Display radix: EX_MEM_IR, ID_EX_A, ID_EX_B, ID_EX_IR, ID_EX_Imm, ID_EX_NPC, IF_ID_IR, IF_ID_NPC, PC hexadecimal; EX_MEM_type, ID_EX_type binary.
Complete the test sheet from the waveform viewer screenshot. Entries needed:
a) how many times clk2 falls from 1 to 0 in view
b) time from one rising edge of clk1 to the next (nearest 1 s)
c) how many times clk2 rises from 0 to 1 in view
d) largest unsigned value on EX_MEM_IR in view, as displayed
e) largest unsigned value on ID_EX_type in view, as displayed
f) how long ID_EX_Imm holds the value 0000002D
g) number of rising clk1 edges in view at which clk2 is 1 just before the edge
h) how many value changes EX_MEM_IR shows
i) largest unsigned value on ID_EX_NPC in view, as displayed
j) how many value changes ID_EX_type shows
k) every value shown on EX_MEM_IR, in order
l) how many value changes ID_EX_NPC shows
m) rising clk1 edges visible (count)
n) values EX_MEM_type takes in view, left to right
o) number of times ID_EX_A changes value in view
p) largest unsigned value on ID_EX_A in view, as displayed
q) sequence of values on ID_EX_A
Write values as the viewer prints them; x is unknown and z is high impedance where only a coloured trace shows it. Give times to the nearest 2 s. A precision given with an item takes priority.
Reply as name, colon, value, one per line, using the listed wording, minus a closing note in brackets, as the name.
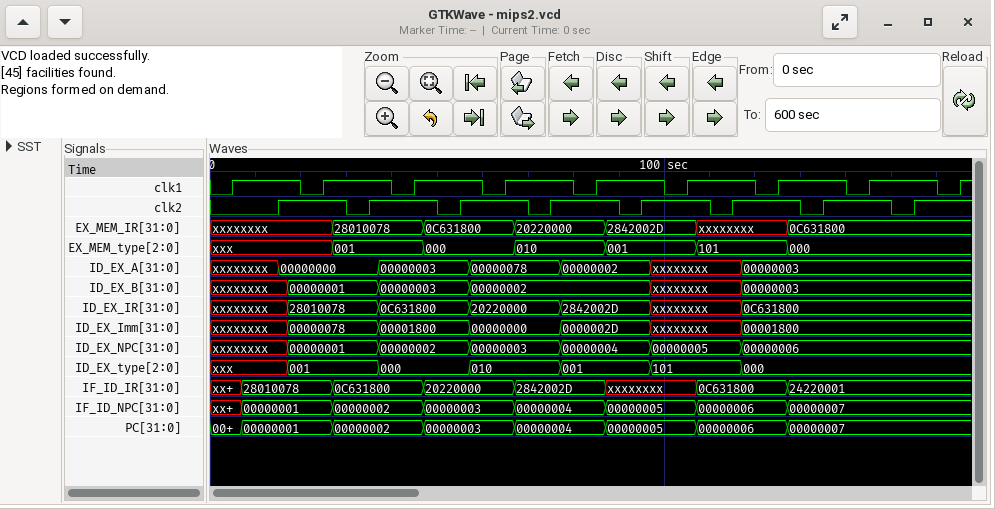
how many times clk2 falls from 1 to 0 in view: 7
time from one rising edge of clk1 to the next: 20 s
how many times clk2 rises from 0 to 1 in view: 8
largest unsigned value on EX_MEM_IR in view, as displayed: 2842002D
largest unsigned value on ID_EX_type in view, as displayed: 101
how long ID_EX_Imm holds the value 0000002D: 20 s
number of rising clk1 edges in view at which clk2 is 1 just before the edge: 8
how many value changes EX_MEM_IR shows: 6
largest unsigned value on ID_EX_NPC in view, as displayed: 00000006
how many value changes ID_EX_type shows: 6
every value shown on EX_MEM_IR, in order: xxxxxxxx, 28010078, 0C631800, 20220000, 2842002D, xxxxxxxx, 0C631800
how many value changes ID_EX_NPC shows: 6
rising clk1 edges visible: 9
values EX_MEM_type takes in view, left to right: xxx, 001, 000, 010, 001, 101, 000
number of times ID_EX_A changes value in view: 6
largest unsigned value on ID_EX_A in view, as displayed: 00000078
sequence of values on ID_EX_A: xxxxxxxx, 00000000, 00000003, 00000078, 00000002, xxxxxxxx, 00000003
